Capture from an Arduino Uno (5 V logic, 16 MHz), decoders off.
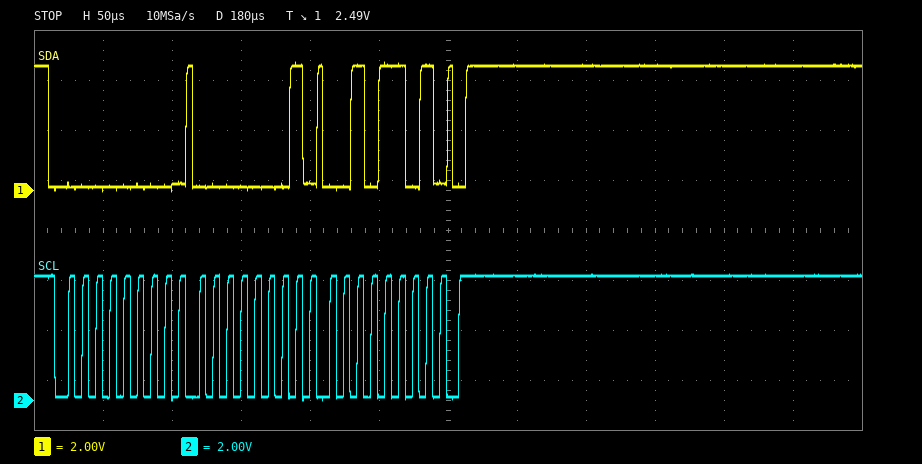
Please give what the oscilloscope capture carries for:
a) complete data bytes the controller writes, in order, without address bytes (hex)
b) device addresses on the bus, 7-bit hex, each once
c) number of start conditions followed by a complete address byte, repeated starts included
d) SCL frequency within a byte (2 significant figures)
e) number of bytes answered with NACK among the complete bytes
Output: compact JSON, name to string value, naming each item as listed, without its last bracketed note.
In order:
{"complete data bytes the controller writes, in order, without address bytes": "01 2D", "device addresses on the bus, 7-bit hex, each once": "0x00", "number of start conditions followed by a complete address byte, repeated starts included": "1", "SCL frequency within a byte": "100 kHz", "number of bytes answered with NACK among the complete bytes": "0"}
